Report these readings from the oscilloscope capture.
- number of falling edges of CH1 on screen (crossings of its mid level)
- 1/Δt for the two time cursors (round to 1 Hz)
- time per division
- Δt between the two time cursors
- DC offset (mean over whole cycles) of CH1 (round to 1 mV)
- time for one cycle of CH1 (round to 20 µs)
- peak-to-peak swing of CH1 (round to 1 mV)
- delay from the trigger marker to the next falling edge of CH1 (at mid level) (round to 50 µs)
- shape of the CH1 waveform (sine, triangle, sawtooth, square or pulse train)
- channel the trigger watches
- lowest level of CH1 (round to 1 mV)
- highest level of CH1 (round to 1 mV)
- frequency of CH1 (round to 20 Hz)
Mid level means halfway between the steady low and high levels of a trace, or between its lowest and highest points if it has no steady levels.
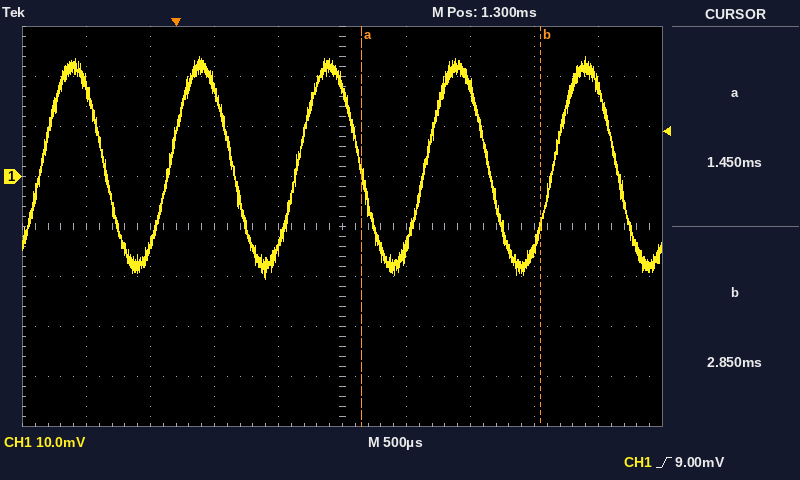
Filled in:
5
714 Hz
500 µs
1.40 ms
2 mV
1.00 ms
44 mV
450 µs
sine
CH1
-20 mV
24 mV
1.00 kHz
